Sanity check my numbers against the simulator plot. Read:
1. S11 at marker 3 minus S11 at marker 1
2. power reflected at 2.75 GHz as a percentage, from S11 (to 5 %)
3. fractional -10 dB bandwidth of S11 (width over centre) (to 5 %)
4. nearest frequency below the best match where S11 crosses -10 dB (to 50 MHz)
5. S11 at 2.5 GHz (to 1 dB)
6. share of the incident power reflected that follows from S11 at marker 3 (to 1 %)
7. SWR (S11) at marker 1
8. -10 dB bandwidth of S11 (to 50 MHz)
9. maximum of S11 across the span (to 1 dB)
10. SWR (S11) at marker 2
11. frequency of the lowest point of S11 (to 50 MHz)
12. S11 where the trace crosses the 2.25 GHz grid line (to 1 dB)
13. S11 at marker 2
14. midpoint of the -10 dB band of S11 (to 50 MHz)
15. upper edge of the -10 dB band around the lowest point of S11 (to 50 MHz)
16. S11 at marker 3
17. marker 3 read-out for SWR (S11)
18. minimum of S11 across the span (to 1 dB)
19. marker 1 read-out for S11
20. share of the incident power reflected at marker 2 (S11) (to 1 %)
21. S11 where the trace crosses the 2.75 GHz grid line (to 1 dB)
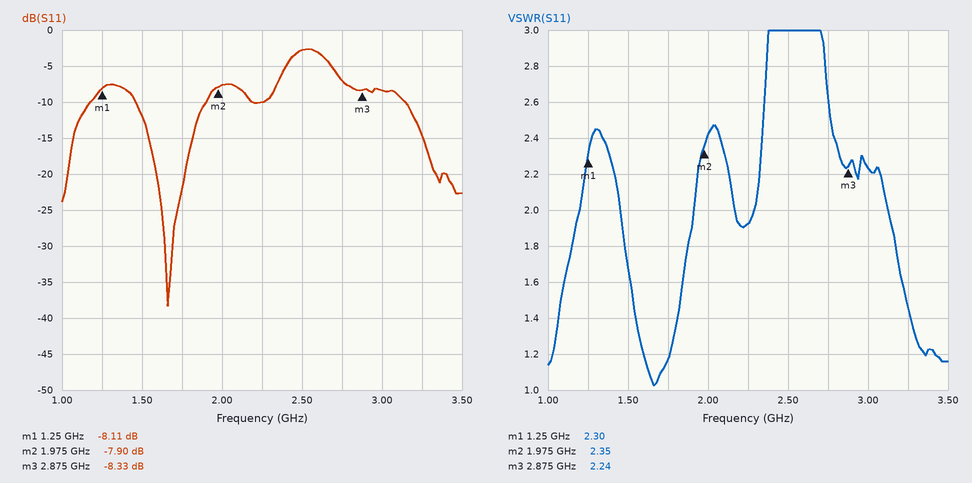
-0.22 dB
20 %
25 %
1.45 GHz
-3 dB
15 %
2.30
450 MHz
-3 dB
2.35
1.65 GHz
-10 dB
-7.90 dB
1.70 GHz
1.90 GHz
-8.33 dB
2.24
-38 dB
-8.11 dB
16 %
-7 dB
